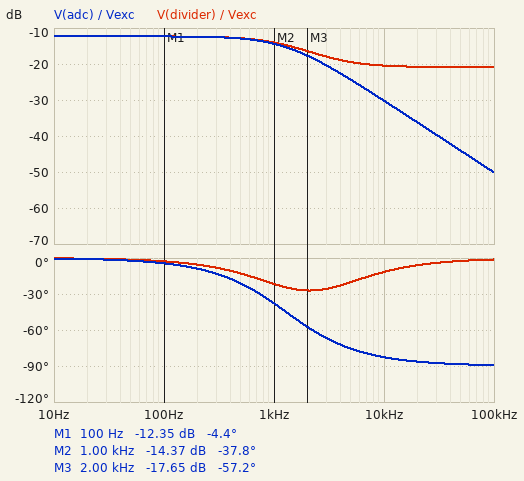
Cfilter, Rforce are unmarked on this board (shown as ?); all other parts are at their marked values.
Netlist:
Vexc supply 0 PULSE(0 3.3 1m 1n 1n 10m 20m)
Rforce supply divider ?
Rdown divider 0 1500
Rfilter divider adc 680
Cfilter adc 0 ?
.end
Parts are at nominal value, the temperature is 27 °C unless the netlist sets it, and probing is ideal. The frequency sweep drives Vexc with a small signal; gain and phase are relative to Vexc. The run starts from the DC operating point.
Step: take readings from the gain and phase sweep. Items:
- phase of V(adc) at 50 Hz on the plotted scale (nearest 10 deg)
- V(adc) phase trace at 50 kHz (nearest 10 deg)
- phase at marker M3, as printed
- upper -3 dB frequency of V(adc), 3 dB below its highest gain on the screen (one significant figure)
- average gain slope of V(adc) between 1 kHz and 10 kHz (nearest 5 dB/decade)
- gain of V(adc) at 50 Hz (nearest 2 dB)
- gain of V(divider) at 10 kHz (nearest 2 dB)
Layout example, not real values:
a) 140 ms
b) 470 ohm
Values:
a) 0 deg
b) -90 deg
c) -57.2 deg
d) 1 kHz
e) -15 dB/decade
f) -12 dB
g) -20 dB
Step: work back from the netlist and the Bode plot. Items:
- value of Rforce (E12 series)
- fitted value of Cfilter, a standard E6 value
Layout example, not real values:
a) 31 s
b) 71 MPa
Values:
a) 4.7 kΩ
b) 68 nF
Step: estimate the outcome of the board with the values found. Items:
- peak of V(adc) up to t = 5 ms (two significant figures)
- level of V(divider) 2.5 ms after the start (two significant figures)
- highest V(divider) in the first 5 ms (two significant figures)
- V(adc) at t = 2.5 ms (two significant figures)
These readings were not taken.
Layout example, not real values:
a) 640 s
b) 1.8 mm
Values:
a) 800 mV
b) 800 mV
c) 800 mV
d) 800 mV
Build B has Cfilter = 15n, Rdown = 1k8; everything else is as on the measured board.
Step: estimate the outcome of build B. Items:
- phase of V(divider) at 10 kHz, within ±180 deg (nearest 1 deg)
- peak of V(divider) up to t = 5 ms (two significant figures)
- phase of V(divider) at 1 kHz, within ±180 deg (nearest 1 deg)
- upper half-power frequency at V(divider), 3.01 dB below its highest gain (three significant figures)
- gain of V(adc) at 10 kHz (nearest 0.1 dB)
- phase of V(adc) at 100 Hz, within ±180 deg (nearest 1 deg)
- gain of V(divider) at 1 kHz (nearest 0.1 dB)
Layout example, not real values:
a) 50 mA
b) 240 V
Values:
a) -29 deg
b) 910 mV
c) -7 deg
d) 6.12 kHz
e) -17.7 dB
f) -1 deg
g) -11.3 dB
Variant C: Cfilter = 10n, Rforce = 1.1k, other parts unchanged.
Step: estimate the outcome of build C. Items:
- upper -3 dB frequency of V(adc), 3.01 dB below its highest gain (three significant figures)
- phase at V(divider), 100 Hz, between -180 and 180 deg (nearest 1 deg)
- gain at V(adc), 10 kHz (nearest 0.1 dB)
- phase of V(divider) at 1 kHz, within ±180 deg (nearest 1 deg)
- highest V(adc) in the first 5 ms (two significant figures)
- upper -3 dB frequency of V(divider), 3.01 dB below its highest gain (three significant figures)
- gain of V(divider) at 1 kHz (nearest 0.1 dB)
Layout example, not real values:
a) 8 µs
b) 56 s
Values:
a) 12.1 kHz
b) 0 deg
c) -7.0 dB
d) -2 deg
e) 1.9 V
f) 17.8 kHz
g) -4.8 dB
